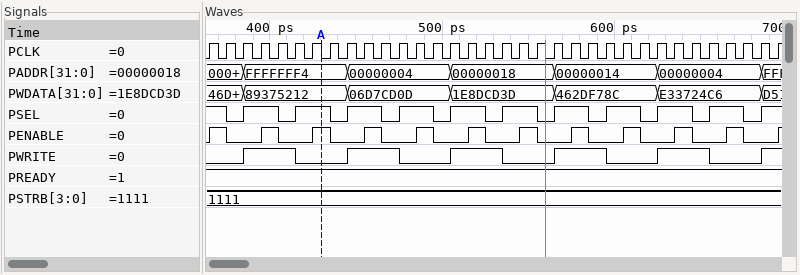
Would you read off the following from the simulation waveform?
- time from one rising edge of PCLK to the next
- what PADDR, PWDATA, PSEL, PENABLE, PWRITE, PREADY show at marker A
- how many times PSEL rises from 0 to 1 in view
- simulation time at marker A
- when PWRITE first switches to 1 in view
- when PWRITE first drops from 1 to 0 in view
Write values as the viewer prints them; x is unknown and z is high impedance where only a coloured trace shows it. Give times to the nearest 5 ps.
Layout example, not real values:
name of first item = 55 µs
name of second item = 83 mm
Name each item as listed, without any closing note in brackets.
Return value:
time from one rising edge of PCLK to the next = 10 ps
what PADDR, PWDATA, PSEL, PENABLE, PWRITE, PREADY show at marker A = PADDR=FFFFFFF4, PWDATA=89375212, PSEL=1, PENABLE=1, PWRITE=0, PREADY=1
how many times PSEL rises from 0 to 1 in view = 11
simulation time at marker A = 430 ps
when PWRITE first switches to 1 in view = 385 ps
when PWRITE first drops from 1 to 0 in view = 415 ps
